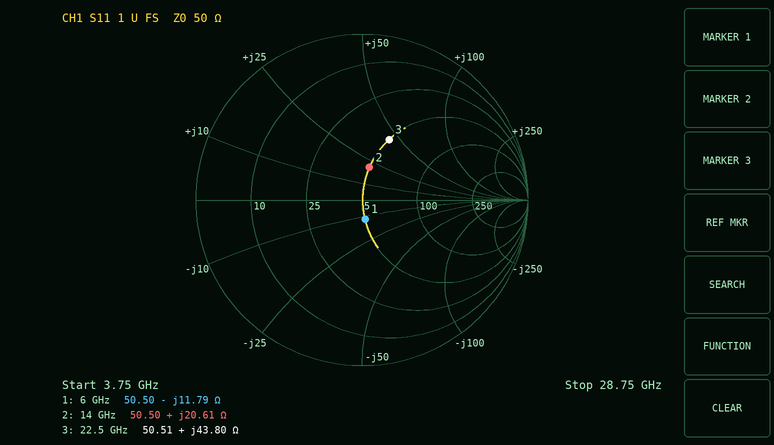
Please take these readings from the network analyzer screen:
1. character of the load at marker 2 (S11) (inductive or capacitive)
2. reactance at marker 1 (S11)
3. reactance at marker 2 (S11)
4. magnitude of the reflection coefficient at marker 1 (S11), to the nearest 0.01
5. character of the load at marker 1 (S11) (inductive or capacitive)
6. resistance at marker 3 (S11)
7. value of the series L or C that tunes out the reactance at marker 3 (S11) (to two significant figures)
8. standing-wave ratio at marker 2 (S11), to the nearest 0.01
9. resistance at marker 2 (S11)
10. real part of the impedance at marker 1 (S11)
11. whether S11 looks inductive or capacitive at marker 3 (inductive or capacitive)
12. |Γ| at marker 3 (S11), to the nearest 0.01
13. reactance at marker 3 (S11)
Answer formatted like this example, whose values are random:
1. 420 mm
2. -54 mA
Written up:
1. inductive
2. -11.79 Ω
3. +20.61 Ω
4. 0.12
5. capacitive
6. 50.51 Ω
7. 160 fF
8. 1.50
9. 50.50 Ω
10. 50.50 Ω
11. inductive
12. 0.40
13. +43.80 Ω
